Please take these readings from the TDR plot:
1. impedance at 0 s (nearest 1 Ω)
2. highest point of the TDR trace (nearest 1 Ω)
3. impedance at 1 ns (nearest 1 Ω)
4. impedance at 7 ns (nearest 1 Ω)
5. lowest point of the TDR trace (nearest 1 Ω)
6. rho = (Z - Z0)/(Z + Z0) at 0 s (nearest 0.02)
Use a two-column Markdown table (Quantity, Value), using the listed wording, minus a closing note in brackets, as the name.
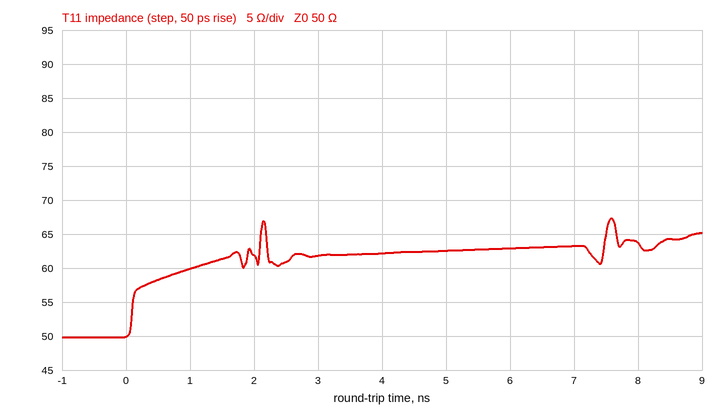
| Quantity | Value |
|---|---|
| impedance at 0 s | 50 Ω |
| highest point of the TDR trace | 67 Ω |
| impedance at 1 ns | 60 Ω |
| impedance at 7 ns | 63 Ω |
| lowest point of the TDR trace | 50 Ω |
| rho = (Z - Z0)/(Z + Z0) at 0 s | 0.00 |
